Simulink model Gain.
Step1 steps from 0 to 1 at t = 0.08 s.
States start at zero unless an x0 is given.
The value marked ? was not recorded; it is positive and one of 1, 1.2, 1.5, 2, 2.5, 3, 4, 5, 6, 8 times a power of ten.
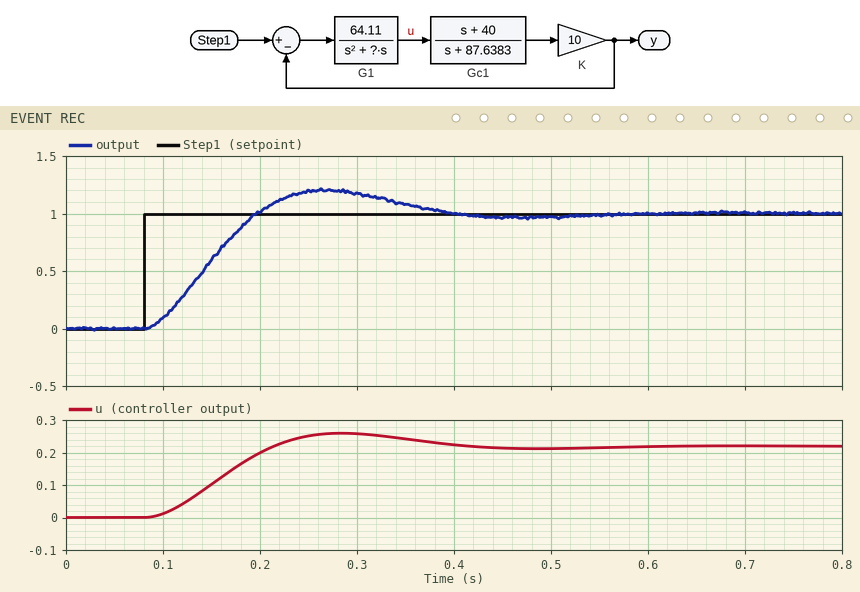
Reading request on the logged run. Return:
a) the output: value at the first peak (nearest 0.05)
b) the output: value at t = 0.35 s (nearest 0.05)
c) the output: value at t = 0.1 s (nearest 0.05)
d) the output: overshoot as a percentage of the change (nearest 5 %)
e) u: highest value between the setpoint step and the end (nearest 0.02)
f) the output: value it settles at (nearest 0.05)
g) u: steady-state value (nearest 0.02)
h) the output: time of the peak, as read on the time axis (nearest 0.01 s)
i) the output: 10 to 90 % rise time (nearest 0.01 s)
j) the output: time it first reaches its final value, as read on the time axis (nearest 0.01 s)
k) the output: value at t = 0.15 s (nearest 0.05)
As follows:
1.20
1.10
0.10
20 %
0.26
1.00
0.22
0.27 s
0.08 s
0.20 s
0.60
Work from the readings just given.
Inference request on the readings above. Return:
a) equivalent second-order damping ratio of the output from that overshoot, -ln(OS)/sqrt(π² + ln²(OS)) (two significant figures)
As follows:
0.46
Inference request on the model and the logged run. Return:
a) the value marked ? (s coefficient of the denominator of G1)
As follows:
12
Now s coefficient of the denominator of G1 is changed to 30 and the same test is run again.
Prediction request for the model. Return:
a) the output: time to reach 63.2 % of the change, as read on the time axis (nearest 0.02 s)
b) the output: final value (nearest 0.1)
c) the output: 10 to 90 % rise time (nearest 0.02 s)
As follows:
0.18 s
1.0
0.18 s
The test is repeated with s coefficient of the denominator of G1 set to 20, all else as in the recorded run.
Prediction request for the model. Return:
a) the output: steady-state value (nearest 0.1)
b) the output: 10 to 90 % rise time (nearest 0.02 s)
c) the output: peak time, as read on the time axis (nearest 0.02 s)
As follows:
1.0
0.12 s
0.32 s
